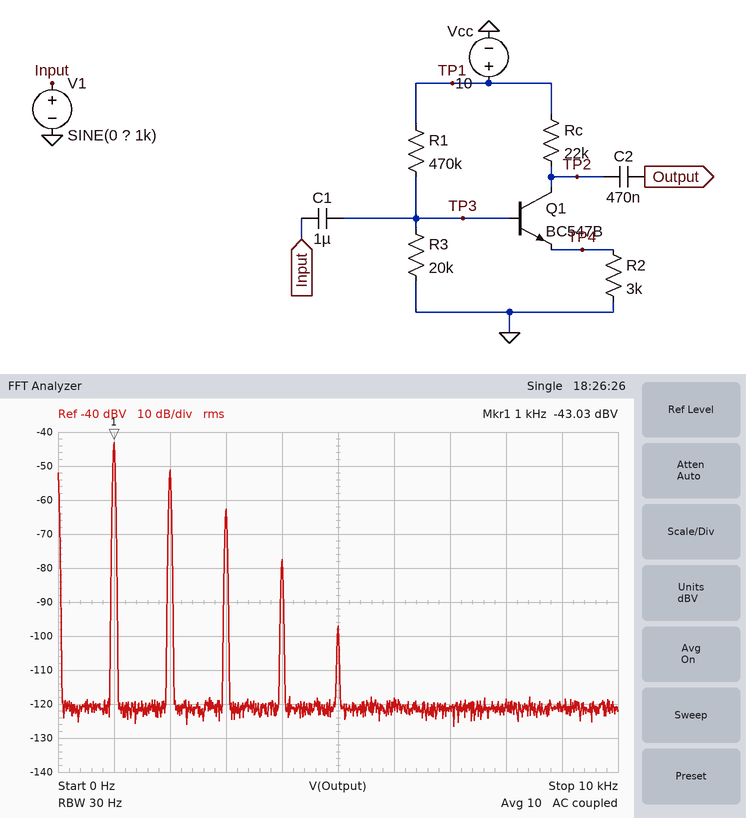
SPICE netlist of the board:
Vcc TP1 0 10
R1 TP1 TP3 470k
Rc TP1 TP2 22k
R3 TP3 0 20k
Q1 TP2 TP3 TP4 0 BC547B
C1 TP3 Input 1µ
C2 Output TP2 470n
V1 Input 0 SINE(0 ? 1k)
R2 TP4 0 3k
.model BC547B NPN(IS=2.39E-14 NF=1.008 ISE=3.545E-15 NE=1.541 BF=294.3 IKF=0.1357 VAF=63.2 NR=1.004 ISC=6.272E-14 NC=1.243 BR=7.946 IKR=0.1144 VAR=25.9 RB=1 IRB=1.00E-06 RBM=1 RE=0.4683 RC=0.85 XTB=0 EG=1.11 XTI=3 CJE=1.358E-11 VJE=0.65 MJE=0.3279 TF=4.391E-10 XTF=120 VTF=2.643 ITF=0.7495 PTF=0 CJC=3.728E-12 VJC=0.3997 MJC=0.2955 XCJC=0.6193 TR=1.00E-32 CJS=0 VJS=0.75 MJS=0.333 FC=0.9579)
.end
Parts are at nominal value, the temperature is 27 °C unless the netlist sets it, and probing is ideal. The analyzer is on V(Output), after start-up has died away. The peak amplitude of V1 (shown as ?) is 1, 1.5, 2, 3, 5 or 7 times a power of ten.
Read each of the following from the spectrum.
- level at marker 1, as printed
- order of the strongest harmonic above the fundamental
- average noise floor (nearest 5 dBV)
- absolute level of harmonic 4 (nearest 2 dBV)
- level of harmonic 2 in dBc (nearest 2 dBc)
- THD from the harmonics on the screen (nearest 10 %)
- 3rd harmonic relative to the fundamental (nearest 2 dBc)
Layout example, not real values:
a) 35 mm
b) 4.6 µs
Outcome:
a) -43.03 dBV
b) 2
c) -120 dBV
d) -78 dBV
e) -8 dBc
f) 40 %
g) -20 dBc
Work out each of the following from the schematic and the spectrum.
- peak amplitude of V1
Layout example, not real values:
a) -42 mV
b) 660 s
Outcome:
a) 50 mV
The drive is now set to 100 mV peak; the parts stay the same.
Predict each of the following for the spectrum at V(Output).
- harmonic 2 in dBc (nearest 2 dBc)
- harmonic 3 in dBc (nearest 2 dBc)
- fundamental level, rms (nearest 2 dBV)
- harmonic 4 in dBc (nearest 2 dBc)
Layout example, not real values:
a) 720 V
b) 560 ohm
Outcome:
a) -4 dBc
b) -12 dBc
c) -30 dBV
d) -24 dBc
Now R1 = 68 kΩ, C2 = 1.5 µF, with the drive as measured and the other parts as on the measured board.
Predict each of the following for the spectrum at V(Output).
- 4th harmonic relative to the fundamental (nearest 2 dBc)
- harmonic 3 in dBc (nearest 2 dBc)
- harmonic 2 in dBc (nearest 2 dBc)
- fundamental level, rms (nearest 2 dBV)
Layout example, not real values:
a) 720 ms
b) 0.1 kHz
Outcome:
a) -42 dBc
b) -30 dBc
c) -18 dBc
d) -34 dBV
